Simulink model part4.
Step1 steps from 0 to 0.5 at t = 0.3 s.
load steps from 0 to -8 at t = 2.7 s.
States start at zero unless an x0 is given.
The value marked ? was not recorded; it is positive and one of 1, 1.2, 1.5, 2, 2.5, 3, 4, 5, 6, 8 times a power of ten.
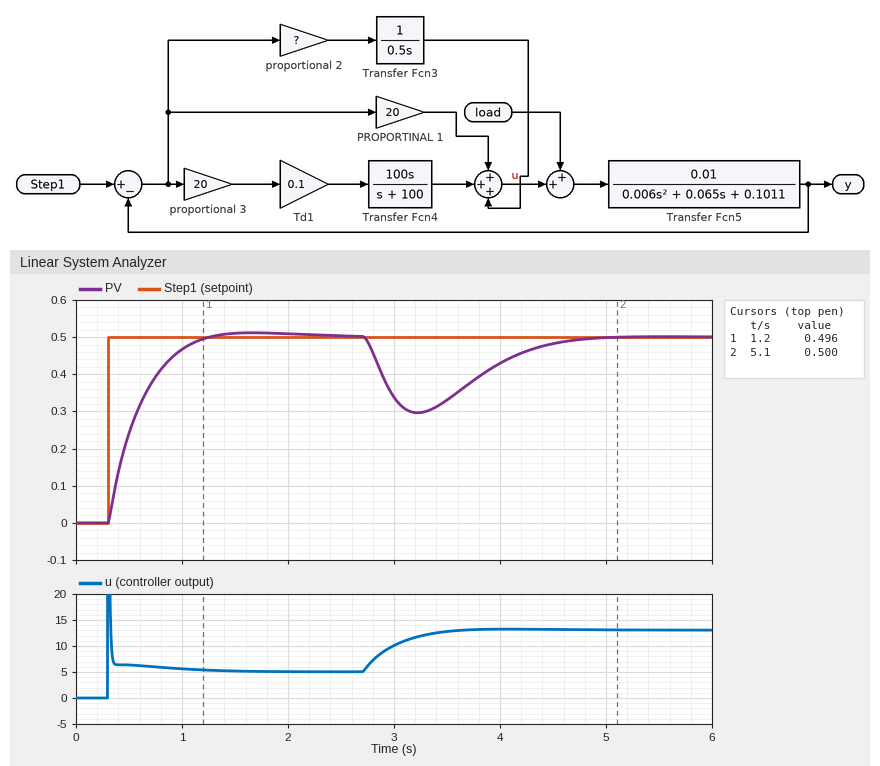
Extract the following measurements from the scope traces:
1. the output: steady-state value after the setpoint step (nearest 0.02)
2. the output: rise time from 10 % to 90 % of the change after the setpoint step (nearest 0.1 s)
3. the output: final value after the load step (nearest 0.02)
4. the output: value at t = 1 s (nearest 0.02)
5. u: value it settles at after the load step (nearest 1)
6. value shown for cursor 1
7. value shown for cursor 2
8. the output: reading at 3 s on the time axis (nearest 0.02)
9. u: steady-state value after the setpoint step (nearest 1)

0.50
0.6 s
0.50
0.46
13
0.496
0.500
0.34
5
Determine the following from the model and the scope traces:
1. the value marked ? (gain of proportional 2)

20
